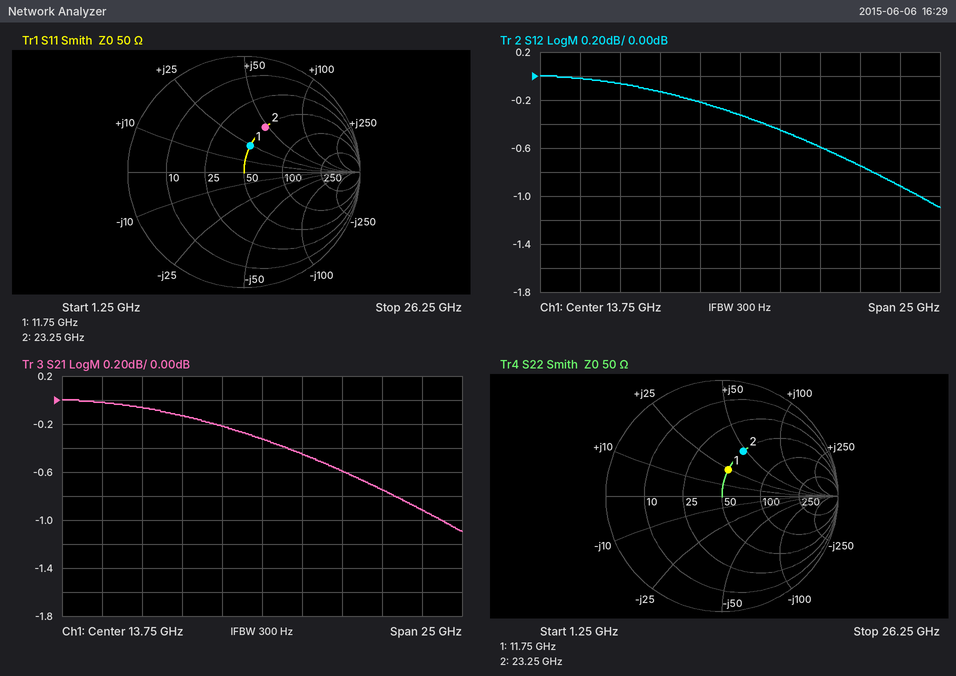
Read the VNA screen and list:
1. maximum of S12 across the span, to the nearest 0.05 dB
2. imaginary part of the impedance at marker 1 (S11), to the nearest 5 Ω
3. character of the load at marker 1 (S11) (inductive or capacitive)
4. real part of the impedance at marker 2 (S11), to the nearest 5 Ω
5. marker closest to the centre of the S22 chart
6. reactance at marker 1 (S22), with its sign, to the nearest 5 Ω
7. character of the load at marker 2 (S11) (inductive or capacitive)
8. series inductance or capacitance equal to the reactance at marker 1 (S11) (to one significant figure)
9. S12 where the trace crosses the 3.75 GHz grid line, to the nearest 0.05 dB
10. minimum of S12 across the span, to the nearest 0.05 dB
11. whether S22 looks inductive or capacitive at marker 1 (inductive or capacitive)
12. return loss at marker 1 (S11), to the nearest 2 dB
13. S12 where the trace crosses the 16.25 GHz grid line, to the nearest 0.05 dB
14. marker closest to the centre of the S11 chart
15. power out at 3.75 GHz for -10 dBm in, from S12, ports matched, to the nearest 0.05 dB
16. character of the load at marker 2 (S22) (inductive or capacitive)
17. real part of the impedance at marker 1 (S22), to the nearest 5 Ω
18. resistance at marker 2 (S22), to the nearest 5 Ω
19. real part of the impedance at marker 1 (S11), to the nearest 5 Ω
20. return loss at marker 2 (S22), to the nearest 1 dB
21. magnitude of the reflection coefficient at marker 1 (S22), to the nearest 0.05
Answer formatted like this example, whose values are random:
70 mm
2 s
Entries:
0.00 dB
+25 Ω
inductive
50 Ω
marker 1
+25 Ω
inductive
300 pH
0.00 dB
-1.10 dB
inductive
12 dB
-0.45 dB
marker 1
-10.00 dBm
inductive
50 Ω
50 Ω
50 Ω
7 dB
0.25
